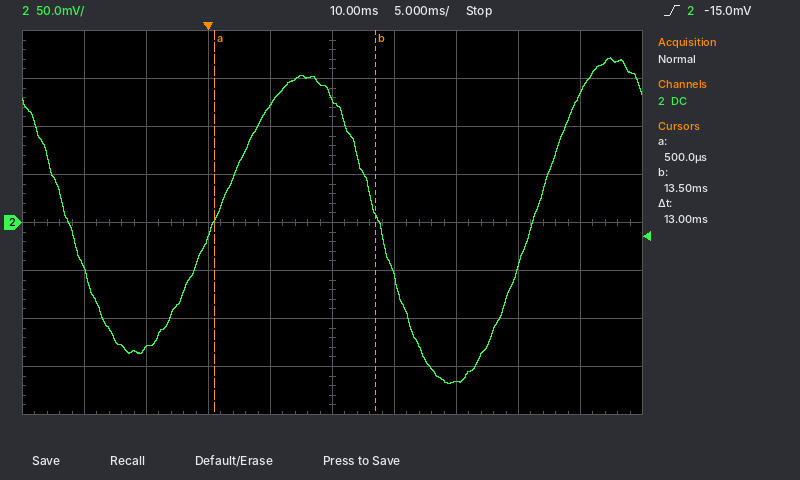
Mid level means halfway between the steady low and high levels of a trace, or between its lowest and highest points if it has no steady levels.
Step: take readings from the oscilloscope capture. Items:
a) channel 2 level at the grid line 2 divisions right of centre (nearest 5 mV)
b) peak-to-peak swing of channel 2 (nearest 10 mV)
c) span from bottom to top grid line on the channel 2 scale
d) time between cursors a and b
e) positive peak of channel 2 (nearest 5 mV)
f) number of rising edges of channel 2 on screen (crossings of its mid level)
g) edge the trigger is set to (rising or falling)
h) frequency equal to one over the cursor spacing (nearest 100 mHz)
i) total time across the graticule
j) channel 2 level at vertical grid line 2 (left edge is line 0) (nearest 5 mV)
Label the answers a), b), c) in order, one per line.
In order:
a) -165 mV
b) 340 mV
c) 400 mV
d) 13 ms
e) 170 mV
f) 2
g) rising
h) 76.9 Hz
i) 50 ms
j) -130 mV
